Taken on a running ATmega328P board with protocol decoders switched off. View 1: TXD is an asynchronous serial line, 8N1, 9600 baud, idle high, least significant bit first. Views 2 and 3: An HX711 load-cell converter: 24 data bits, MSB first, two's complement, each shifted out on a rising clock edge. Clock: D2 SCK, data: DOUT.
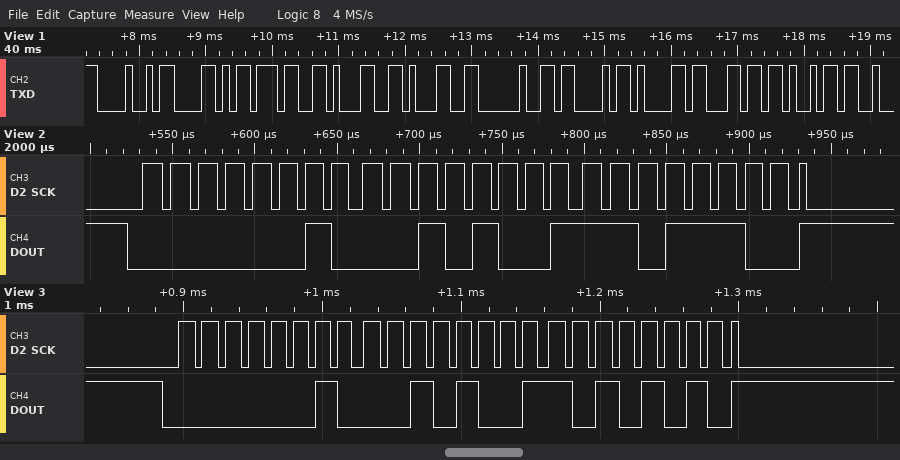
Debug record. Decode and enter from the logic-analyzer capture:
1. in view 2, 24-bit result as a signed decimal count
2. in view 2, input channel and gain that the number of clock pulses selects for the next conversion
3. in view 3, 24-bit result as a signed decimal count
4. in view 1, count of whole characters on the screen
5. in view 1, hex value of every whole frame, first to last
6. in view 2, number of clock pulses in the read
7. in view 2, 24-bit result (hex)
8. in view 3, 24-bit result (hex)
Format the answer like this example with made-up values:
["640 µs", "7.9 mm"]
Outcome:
["141788", "channel A, gain 128", "141738", "10", "48 58 37 31 31 20 43 61 6C 69", "25", "0x0229DC", "0x0229AA"]
